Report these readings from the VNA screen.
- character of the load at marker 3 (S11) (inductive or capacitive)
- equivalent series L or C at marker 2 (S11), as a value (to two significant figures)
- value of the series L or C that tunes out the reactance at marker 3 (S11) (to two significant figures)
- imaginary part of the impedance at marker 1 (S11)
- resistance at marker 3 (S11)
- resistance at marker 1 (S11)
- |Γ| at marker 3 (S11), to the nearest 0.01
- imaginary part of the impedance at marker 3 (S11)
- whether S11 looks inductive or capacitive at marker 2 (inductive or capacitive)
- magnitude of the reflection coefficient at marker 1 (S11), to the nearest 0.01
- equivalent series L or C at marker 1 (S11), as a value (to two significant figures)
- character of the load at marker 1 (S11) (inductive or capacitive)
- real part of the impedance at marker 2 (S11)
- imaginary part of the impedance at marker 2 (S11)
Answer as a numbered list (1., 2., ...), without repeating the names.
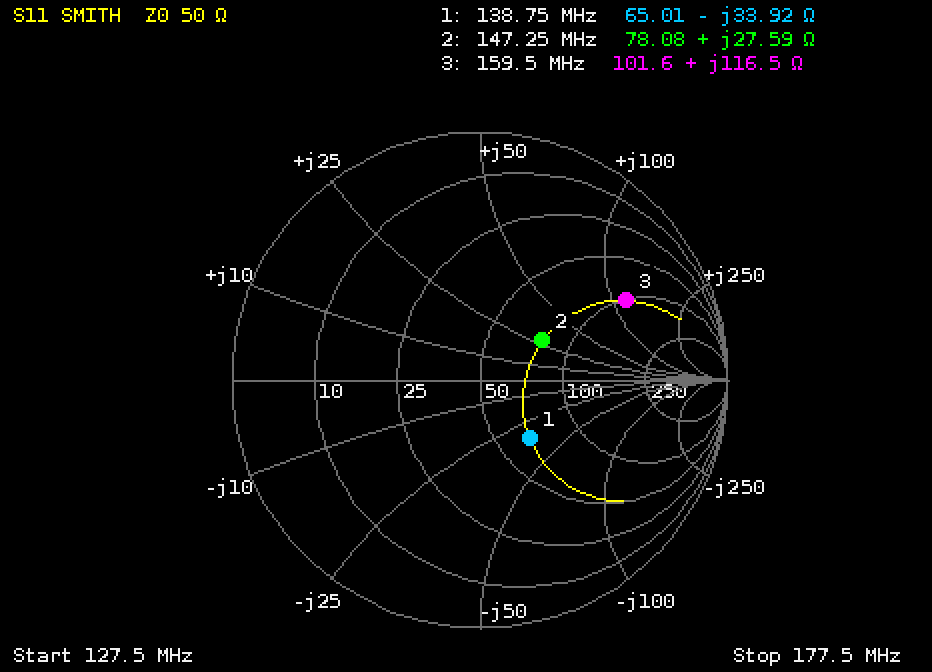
1. inductive
2. 30 nH
3. 8.6 pF
4. -33.92 Ω
5. 101.6 Ω
6. 65.01 Ω
7. 0.67
8. +116.5 Ω
9. inductive
10. 0.31
11. 34 pF
12. capacitive
13. 78.08 Ω
14. +27.59 Ω
